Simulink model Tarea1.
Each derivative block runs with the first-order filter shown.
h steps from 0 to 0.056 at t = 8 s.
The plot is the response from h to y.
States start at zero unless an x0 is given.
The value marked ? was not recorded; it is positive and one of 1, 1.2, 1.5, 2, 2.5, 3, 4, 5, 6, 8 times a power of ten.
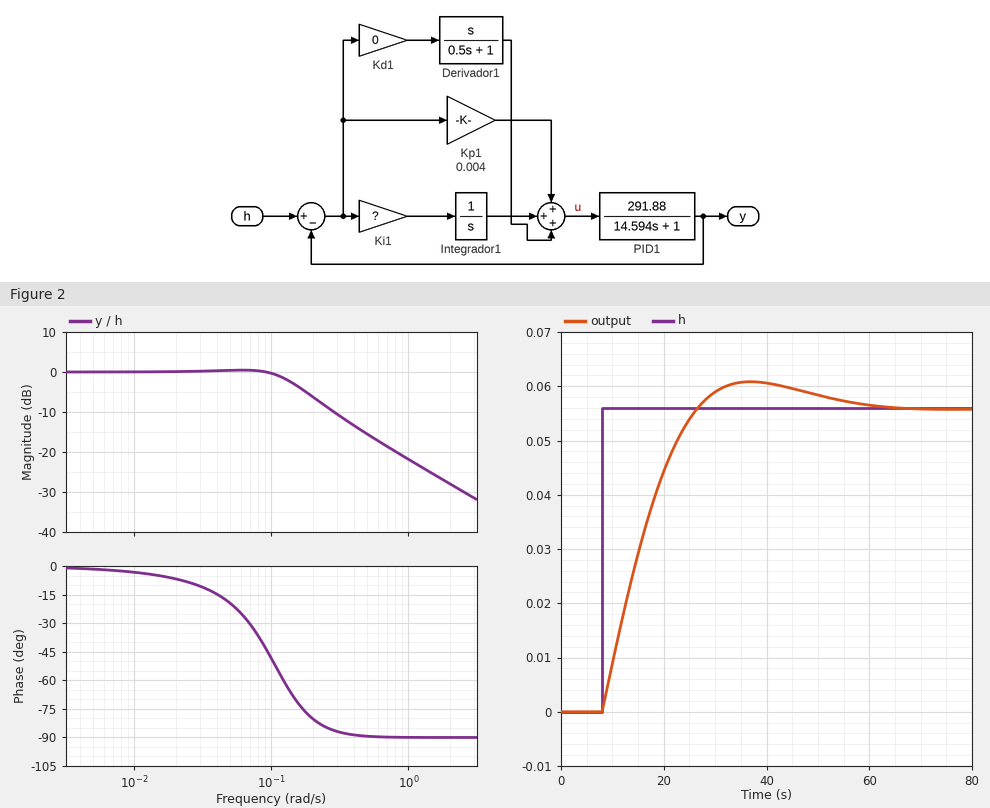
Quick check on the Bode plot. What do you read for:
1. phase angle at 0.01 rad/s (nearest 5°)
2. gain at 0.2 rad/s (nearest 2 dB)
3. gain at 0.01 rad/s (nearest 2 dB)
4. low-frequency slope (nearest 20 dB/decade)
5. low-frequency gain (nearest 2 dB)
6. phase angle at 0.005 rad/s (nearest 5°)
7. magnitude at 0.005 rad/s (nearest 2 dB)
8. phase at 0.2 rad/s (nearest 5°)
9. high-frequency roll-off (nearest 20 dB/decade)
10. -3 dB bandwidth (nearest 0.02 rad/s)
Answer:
-5°
-6 dB
0 dB
0 dB/decade
0 dB
0°
0 dB
-80°
-20 dB/decade
0.14 rad/s
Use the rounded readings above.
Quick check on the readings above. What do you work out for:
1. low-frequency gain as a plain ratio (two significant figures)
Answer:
1.0
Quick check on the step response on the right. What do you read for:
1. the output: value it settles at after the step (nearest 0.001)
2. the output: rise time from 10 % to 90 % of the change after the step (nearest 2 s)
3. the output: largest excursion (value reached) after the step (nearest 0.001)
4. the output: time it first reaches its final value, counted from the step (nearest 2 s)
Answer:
0.056
14 s
0.061
18 s
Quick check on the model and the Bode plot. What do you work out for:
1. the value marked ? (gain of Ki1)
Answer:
0.0006
